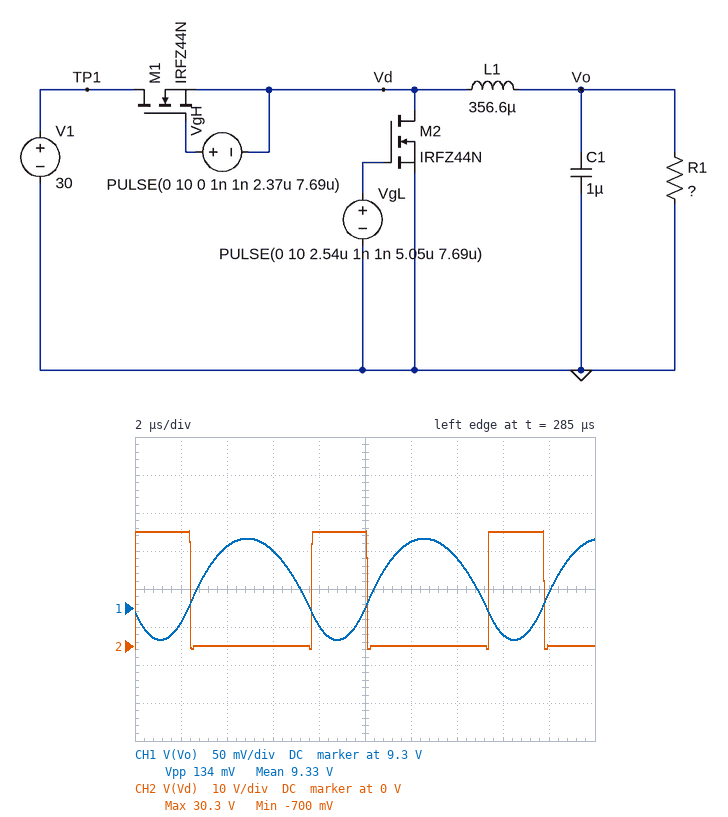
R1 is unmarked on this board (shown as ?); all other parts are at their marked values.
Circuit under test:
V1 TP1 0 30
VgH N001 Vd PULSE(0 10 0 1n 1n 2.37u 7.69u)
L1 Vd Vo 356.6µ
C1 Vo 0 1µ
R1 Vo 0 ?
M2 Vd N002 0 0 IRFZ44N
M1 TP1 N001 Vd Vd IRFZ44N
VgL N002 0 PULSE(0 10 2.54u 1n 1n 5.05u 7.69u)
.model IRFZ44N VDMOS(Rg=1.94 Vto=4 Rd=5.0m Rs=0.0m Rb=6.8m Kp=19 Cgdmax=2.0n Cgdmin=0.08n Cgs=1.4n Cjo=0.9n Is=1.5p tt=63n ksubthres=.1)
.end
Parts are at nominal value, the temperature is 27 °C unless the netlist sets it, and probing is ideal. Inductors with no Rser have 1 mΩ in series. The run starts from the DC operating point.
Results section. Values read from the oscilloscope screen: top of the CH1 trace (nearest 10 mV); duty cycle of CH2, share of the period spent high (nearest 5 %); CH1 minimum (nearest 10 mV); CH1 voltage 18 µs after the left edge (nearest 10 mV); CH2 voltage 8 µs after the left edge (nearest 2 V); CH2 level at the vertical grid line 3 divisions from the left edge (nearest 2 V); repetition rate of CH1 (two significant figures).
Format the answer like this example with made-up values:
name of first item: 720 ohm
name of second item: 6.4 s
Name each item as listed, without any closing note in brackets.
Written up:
top of the CH1 trace: 9.39 V
duty cycle of CH2, share of the period spent high: 30 %
CH1 minimum: 9.26 V
CH1 voltage 18 µs after the left edge: 9.32 V
CH2 voltage 8 µs after the left edge: 30 V
CH2 level at the vertical grid line 3 divisions from the left edge: 0 V
repetition rate of CH1: 130 kHz
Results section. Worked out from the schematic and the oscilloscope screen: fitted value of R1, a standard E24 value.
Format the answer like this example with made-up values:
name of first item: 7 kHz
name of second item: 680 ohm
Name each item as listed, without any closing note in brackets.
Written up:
fitted value of R1, a standard E24 value: 13 Ω
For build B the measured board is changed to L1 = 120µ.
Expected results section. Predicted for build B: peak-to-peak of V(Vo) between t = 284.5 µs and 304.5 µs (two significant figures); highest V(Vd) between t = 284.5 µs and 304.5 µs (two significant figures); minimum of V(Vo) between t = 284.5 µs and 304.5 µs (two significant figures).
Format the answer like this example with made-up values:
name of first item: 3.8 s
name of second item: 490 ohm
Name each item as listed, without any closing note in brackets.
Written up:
peak-to-peak of V(Vo) between t = 284.5 µs and 304.5 µs: 400 mV
highest V(Vd) between t = 284.5 µs and 304.5 µs: 30 V
minimum of V(Vo) between t = 284.5 µs and 304.5 µs: 9.1 V
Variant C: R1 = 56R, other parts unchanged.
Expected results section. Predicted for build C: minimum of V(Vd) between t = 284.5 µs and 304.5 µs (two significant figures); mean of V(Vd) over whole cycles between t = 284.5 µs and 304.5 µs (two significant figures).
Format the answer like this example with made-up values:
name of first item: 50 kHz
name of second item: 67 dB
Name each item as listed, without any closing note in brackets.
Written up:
minimum of V(Vd) between t = 284.5 µs and 304.5 µs: -650 mV
mean of V(Vd) over whole cycles between t = 284.5 µs and 304.5 µs: 9.6 V
